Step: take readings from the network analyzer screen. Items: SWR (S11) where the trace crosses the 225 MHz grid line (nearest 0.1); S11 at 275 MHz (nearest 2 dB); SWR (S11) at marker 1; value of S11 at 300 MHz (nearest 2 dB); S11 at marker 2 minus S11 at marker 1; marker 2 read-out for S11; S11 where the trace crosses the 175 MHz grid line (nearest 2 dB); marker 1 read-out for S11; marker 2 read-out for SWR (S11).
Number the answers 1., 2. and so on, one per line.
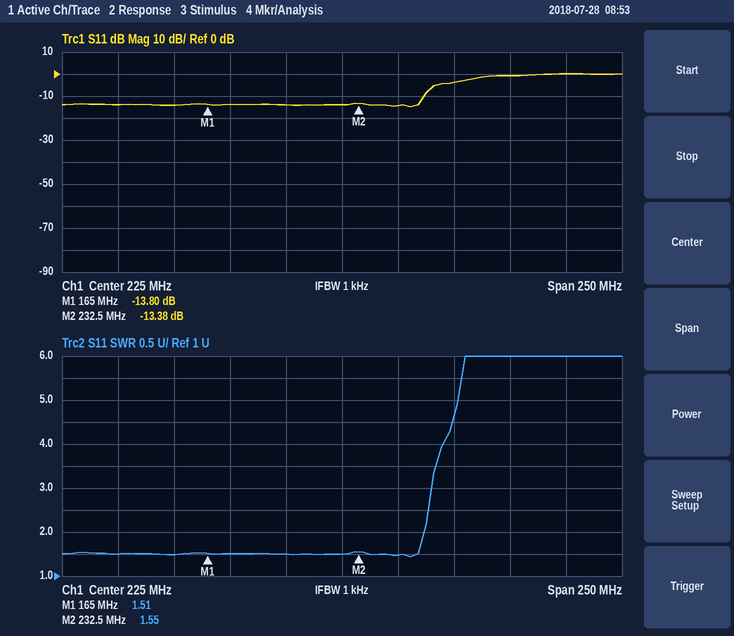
1. 1.5
2. -4 dB
3. 1.51
4. 0 dB
5. 0.42 dB
6. -13.38 dB
7. -14 dB
8. -13.80 dB
9. 1.55
